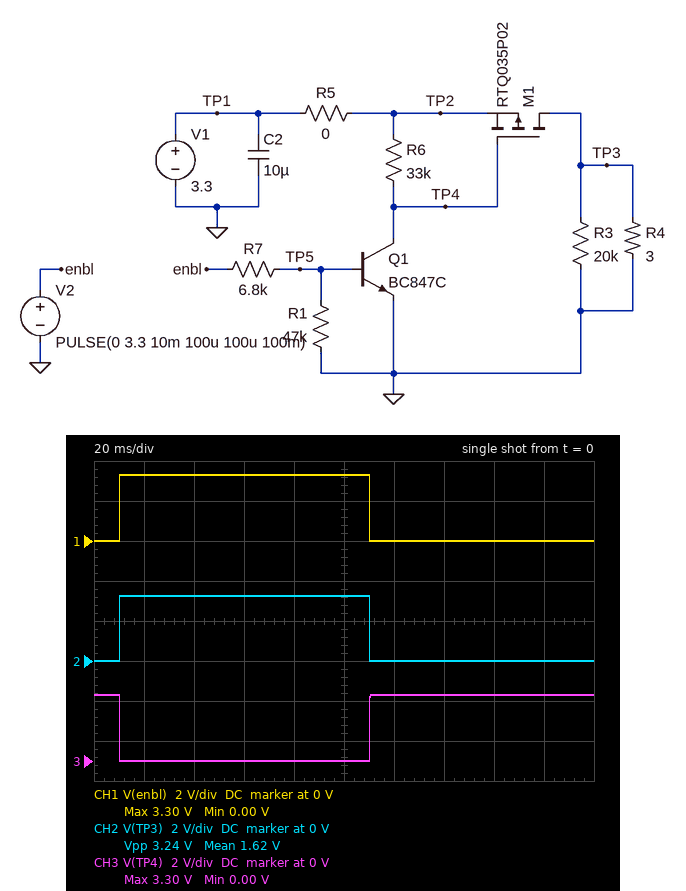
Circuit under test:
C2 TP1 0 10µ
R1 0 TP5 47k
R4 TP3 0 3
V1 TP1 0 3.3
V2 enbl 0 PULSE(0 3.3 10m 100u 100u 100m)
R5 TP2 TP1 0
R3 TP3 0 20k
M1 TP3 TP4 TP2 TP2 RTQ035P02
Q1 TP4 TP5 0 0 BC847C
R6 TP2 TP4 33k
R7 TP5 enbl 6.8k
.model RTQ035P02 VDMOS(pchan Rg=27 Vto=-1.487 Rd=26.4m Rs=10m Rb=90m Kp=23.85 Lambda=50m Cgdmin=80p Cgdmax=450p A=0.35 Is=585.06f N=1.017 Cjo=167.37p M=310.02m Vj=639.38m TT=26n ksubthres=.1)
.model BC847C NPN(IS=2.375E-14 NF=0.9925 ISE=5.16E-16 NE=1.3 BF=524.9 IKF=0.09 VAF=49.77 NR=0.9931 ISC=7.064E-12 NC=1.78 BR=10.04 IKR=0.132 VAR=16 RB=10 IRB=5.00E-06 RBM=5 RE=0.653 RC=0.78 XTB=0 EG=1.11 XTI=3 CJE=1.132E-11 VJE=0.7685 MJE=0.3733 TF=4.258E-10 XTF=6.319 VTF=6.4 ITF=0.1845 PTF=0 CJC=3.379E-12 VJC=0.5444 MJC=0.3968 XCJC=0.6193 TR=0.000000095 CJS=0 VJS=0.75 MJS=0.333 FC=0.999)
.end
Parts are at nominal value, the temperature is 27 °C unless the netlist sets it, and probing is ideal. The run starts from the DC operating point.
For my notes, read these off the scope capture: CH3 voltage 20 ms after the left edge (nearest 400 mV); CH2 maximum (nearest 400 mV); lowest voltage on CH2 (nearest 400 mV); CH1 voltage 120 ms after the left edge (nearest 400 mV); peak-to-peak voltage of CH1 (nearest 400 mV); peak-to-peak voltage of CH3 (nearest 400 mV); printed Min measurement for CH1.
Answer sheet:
0 V
3.2 V
0 V
0 V
3.2 V
3.2 V
0.00 V
